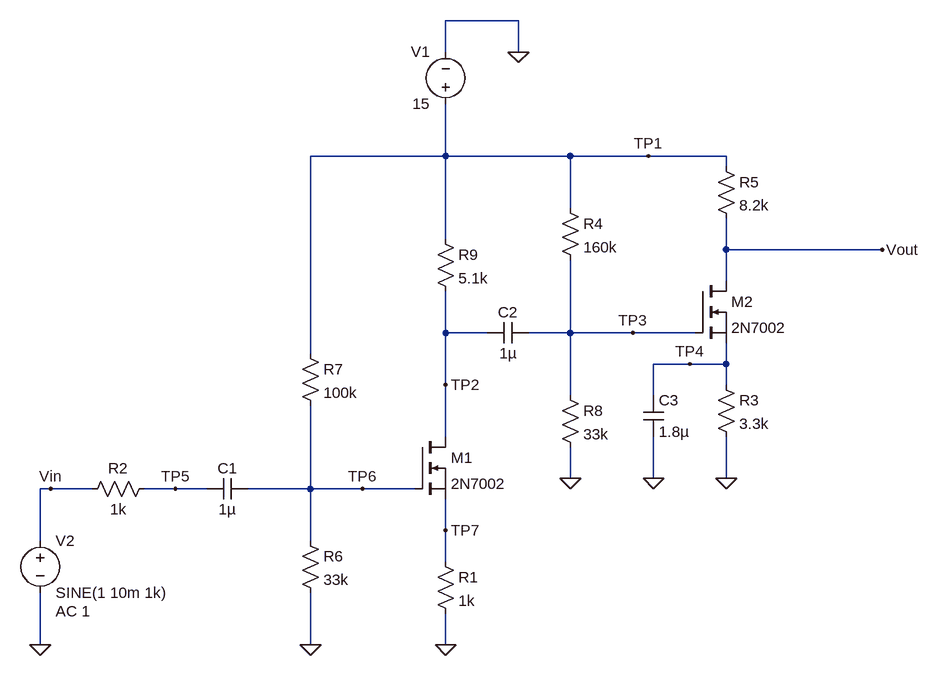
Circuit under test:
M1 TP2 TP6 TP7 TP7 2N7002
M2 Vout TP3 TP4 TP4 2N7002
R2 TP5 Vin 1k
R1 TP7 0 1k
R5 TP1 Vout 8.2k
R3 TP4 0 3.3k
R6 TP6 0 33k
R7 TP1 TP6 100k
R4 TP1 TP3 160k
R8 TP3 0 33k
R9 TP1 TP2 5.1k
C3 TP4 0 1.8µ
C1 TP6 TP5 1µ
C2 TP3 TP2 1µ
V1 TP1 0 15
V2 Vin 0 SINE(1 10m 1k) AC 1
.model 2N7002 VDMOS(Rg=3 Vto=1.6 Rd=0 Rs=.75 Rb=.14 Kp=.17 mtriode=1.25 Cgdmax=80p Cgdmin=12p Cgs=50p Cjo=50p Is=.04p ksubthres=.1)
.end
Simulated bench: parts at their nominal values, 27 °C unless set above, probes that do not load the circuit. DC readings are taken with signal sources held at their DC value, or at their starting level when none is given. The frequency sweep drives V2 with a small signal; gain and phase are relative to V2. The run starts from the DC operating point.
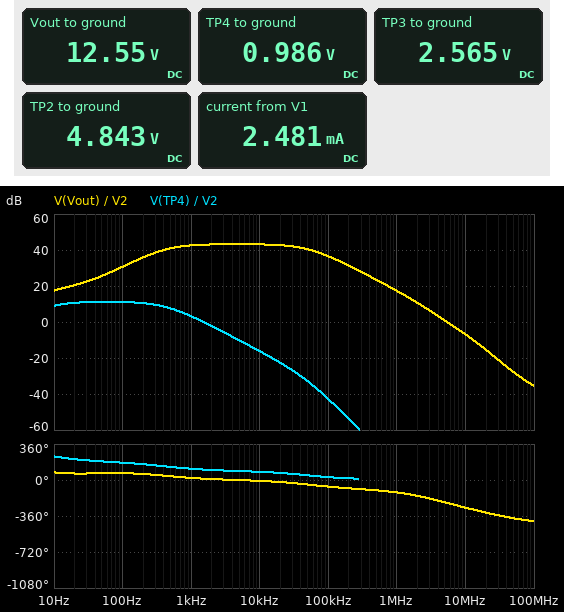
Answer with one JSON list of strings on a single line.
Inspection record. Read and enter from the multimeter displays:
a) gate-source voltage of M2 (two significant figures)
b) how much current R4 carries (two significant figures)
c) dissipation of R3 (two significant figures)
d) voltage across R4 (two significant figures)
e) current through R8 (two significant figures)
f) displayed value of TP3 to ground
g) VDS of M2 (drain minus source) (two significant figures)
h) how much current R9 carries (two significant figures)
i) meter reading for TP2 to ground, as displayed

["1.6 V", "78 µA", "290 µW", "12 V", "78 µA", "2.565 V", "12 V", "2.0 mA", "4.843 V"]
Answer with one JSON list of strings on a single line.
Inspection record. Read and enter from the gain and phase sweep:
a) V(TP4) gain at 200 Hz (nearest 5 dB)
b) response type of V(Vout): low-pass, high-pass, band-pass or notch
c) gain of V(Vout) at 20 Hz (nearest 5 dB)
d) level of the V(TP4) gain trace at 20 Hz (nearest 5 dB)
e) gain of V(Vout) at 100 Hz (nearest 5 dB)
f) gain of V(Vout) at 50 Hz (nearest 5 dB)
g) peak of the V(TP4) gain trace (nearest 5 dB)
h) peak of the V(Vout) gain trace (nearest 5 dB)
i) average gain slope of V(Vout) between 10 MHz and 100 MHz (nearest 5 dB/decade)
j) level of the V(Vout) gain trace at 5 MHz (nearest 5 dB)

["10 dB", "band-pass", "20 dB", "10 dB", "30 dB", "25 dB", "10 dB", "45 dB", "-30 dB/decade", "0 dB"]
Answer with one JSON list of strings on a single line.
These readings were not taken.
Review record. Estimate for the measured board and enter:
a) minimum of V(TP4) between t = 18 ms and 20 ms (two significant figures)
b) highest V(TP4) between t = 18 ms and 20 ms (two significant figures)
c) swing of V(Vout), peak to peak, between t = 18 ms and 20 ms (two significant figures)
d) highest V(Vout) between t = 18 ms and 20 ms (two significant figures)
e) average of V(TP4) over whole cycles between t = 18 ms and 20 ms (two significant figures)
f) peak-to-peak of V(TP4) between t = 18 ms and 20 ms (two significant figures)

["980 mV", "1.0 V", "2.6 V", "14 V", "990 mV", "28 mV"]
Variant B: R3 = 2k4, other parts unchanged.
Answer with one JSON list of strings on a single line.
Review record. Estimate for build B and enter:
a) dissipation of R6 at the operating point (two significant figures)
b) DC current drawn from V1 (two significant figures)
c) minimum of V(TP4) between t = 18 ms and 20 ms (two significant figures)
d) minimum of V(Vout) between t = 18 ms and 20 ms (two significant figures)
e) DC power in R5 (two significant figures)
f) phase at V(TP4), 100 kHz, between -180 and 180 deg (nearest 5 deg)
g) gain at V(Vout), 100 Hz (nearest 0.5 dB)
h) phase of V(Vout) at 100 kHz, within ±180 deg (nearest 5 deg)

["420 µW", "2.6 mA", "950 mV", "9.9 V", "1.3 mW", "25 deg", "31.0 dB", "-70 deg"]
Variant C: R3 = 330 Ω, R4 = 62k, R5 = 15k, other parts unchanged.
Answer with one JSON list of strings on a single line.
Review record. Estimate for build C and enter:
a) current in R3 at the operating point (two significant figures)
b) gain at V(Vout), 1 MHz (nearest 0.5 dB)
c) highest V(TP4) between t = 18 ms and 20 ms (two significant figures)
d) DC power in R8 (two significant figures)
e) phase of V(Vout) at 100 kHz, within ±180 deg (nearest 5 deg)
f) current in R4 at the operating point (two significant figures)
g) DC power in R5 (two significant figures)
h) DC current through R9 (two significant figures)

["980 µA", "-59.5 dB", "320 mV", "820 µW", "-50 deg", "160 µA", "14 mW", "2.0 mA"]
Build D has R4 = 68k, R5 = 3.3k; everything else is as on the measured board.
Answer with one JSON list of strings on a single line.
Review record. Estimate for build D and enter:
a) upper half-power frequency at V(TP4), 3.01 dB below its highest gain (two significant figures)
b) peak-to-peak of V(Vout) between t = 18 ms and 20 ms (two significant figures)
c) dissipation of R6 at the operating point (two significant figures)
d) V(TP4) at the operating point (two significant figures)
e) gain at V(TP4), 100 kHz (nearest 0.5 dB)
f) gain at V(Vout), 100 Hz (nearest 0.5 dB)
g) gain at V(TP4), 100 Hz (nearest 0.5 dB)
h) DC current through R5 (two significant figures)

["1.1 kHz", "2.0 V", "420 µW", "3.2 V", "-35.0 dB", "23.0 dB", "11.5 dB", "980 µA"]
